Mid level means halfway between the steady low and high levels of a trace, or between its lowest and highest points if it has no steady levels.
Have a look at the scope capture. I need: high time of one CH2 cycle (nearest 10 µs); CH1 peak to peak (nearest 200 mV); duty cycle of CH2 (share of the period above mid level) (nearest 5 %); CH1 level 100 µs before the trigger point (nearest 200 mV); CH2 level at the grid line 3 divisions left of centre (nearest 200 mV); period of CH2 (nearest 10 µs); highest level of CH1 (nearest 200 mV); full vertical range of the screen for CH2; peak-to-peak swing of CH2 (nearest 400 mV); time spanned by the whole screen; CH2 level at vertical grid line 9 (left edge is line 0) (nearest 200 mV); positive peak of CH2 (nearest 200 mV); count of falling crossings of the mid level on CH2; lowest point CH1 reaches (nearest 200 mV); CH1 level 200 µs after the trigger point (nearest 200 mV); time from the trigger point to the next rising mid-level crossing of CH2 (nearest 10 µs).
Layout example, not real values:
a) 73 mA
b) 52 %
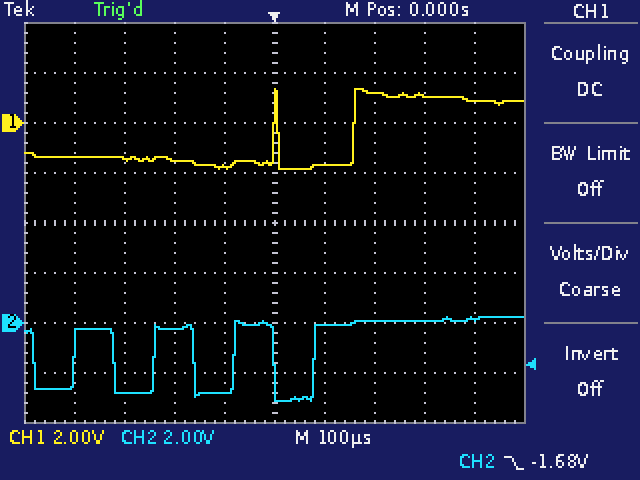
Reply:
a) 80 µs
b) 3.2 V
c) 50 %
d) -1.8 V
e) -2.8 V
f) 160 µs
g) 1.4 V
h) 16 V
i) 3.2 V
j) 1 ms
k) 200 mV
l) 200 mV
m) 4
n) -1.8 V
o) 1.2 V
p) 80 µs
